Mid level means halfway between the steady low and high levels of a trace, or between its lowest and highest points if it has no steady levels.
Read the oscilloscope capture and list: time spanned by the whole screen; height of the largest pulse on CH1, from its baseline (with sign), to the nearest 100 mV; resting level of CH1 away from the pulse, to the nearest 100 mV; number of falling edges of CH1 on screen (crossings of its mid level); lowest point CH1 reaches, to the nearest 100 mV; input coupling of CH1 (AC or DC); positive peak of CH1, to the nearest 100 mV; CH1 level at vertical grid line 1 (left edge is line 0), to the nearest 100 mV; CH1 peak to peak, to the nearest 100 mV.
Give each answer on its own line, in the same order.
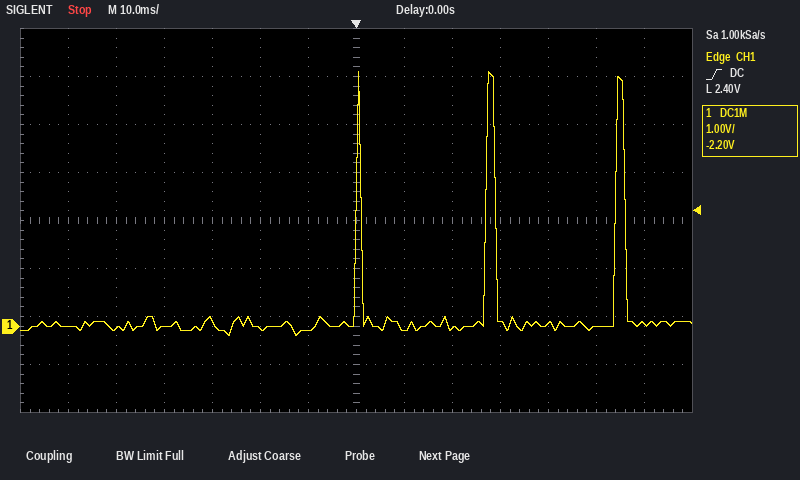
140 ms
+5.3 V
0.0 V
3
-200 mV
DC
5.3 V
0.0 V
5.5 V
